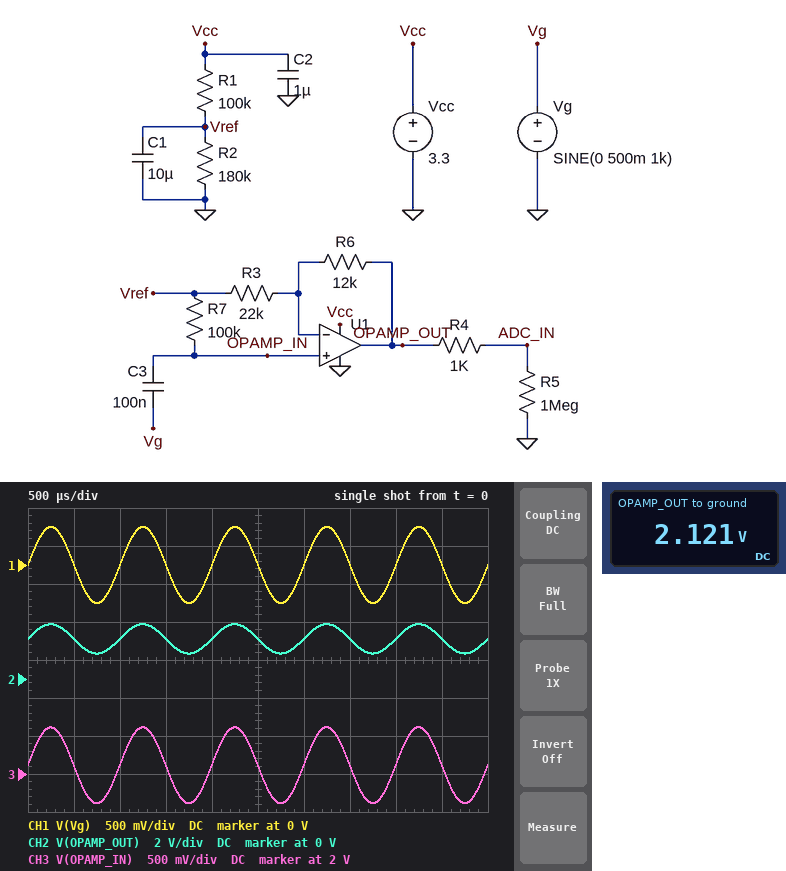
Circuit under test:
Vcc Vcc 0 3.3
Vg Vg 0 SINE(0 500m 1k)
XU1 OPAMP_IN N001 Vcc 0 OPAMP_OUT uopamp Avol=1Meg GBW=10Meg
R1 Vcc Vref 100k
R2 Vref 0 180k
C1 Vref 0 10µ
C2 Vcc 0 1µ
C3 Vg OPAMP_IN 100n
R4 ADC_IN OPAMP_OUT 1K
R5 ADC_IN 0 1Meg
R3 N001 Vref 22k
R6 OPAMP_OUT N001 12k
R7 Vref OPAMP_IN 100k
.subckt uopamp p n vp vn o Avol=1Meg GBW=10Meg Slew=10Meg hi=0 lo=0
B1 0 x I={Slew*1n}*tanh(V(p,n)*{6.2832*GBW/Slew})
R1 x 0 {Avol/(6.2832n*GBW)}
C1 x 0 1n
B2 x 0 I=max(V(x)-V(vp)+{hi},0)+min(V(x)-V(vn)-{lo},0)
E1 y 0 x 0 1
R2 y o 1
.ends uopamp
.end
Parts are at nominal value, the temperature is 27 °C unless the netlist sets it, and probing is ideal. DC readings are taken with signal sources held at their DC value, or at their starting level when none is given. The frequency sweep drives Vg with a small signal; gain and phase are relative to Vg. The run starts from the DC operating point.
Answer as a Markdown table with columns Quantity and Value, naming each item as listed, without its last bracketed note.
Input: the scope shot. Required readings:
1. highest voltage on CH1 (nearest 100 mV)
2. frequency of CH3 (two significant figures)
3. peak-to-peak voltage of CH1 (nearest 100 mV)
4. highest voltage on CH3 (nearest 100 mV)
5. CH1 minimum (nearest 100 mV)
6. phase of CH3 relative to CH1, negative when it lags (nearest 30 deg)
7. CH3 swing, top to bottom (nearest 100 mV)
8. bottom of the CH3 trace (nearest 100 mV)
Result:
| Quantity | Value |
|---|---|
| highest voltage on CH1 | 500 mV |
| frequency of CH3 | 1.0 kHz |
| peak-to-peak voltage of CH1 | 1.0 V |
| highest voltage on CH3 | 2.6 V |
| CH1 minimum | -500 mV |
| phase of CH3 relative to CH1, negative when it lags | 0 deg |
| CH3 swing, top to bottom | 1.0 V |
| bottom of the CH3 trace | 1.6 V |
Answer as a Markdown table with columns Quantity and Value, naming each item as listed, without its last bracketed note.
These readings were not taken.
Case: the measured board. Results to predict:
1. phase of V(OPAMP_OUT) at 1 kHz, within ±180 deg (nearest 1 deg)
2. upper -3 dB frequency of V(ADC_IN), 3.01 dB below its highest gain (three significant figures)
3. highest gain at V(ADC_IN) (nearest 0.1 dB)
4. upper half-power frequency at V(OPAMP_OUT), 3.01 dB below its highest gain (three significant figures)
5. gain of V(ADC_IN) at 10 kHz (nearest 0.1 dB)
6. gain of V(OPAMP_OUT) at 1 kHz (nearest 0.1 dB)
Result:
| Quantity | Value |
|---|---|
| phase of V(OPAMP_OUT) at 1 kHz, within ±180 deg | 1 deg |
| upper -3 dB frequency of V(ADC_IN), 3.01 dB below its highest gain | 6.47 MHz |
| highest gain at V(ADC_IN) | 3.8 dB |
| upper half-power frequency at V(OPAMP_OUT), 3.01 dB below its highest gain | 6.47 MHz |
| gain of V(ADC_IN) at 10 kHz | 3.8 dB |
| gain of V(OPAMP_OUT) at 1 kHz | 3.8 dB |
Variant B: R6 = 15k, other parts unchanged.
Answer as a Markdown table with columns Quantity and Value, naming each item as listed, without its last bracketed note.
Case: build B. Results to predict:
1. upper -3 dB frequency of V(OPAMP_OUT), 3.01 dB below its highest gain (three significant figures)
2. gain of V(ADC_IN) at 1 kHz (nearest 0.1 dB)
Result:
| Quantity | Value |
|---|---|
| upper -3 dB frequency of V(OPAMP_OUT), 3.01 dB below its highest gain | 5.95 MHz |
| gain of V(ADC_IN) at 1 kHz | 4.5 dB |
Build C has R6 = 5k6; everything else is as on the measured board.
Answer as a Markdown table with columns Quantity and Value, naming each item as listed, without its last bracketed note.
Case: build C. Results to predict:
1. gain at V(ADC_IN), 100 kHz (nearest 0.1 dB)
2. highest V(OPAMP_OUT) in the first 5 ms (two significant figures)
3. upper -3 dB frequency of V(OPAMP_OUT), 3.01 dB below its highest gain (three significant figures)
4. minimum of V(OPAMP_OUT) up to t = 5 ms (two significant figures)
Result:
| Quantity | Value |
|---|---|
| gain at V(ADC_IN), 100 kHz | 2.0 dB |
| highest V(OPAMP_OUT) in the first 5 ms | 2.7 V |
| upper -3 dB frequency of V(OPAMP_OUT), 3.01 dB below its highest gain | 7.97 MHz |
| minimum of V(OPAMP_OUT) up to t = 5 ms | 1.5 V |
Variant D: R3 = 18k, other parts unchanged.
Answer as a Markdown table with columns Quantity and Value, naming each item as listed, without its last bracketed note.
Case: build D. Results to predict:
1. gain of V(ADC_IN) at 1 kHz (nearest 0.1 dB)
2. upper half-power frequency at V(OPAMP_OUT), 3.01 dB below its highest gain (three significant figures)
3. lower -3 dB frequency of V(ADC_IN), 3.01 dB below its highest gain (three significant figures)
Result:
| Quantity | Value |
|---|---|
| gain of V(ADC_IN) at 1 kHz | 4.4 dB |
| upper half-power frequency at V(OPAMP_OUT), 3.01 dB below its highest gain | 6.00 MHz |
| lower -3 dB frequency of V(ADC_IN), 3.01 dB below its highest gain | 16.9 Hz |
